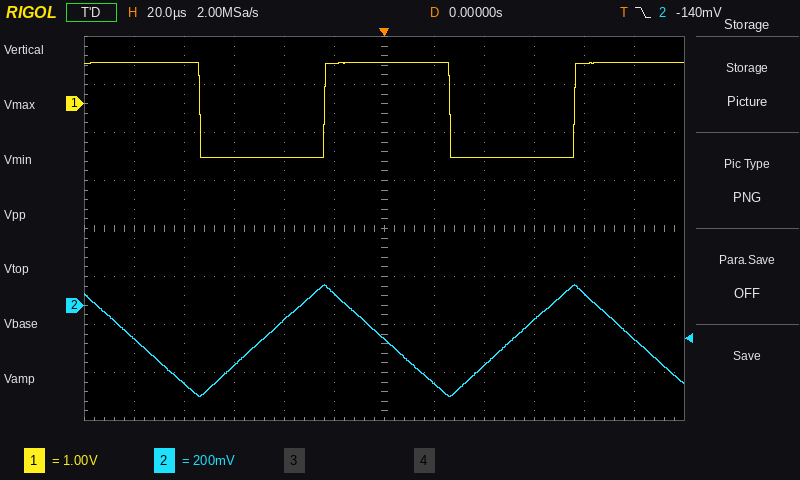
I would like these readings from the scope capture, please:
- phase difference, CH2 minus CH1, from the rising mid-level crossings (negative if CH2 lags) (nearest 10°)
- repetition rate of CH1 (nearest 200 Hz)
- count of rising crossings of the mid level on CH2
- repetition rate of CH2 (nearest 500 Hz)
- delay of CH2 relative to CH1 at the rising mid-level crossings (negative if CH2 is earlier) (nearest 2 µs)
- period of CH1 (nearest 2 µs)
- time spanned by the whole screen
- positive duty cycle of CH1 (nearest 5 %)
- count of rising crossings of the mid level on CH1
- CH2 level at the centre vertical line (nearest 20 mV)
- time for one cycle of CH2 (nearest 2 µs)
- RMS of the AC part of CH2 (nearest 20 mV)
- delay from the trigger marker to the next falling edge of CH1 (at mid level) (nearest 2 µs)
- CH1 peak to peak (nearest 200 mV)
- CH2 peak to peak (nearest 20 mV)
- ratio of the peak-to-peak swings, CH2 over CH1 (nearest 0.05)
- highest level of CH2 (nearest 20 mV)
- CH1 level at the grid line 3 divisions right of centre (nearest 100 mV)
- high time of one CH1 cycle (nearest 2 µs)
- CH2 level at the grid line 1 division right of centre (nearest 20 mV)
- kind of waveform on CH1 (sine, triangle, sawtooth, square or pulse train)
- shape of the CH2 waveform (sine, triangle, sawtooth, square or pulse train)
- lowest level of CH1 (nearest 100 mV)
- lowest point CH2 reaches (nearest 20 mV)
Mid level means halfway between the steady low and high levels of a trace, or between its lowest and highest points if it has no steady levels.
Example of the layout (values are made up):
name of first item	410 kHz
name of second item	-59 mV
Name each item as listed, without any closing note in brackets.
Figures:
phase difference, CH2 minus CH1, from the rising mid-level crossings (negative if CH2 lags)	+90°
repetition rate of CH1	10.0 kHz
count of rising crossings of the mid level on CH2	2
repetition rate of CH2	10.0 kHz
delay of CH2 relative to CH1 at the rising mid-level crossings (negative if CH2 is earlier)	-26 µs
period of CH1	100 µs
time spanned by the whole screen	240 µs
positive duty cycle of CH1	50 %
count of rising crossings of the mid level on CH1	2
CH2 level at the centre vertical line	-140 mV
time for one cycle of CH2	100 µs
RMS of the AC part of CH2	140 mV
delay from the trigger marker to the next falling edge of CH1 (at mid level)	26 µs
CH1 peak to peak	2.0 V
CH2 peak to peak	460 mV
ratio of the peak-to-peak swings, CH2 over CH1	0.25
highest level of CH2	80 mV
CH1 level at the grid line 3 divisions right of centre	-1.1 V
high time of one CH1 cycle	50 µs
CH2 level at the grid line 1 division right of centre	-320 mV
kind of waveform on CH1	square
shape of the CH2 waveform	triangle
lowest level of CH1	-1.1 V
lowest point CH2 reaches	-380 mV
